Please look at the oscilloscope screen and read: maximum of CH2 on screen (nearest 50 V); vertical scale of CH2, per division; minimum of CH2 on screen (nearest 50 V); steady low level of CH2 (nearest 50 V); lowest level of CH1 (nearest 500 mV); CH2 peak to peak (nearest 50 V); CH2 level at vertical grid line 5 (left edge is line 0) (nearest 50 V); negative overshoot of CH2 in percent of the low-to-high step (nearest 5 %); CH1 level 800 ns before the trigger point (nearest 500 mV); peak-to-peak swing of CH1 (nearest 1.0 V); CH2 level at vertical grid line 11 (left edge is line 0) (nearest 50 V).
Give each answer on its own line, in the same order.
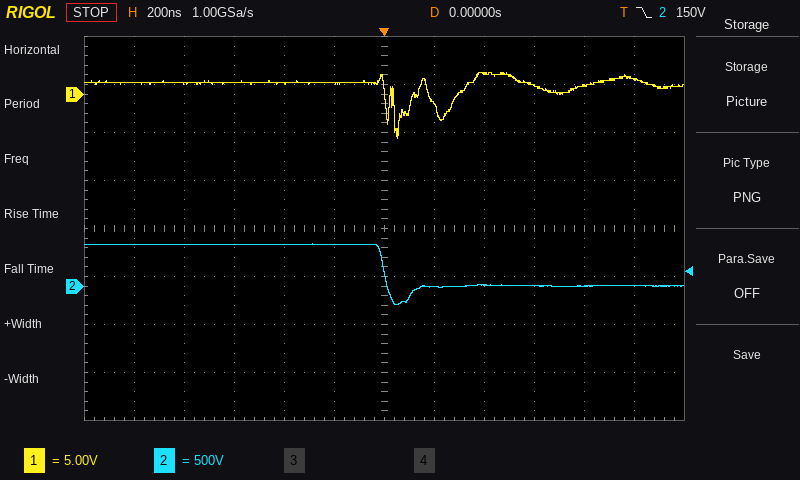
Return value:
450 V
500 V
-200 V
0 V
-4.5 V
650 V
450 V
45 %
1.0 V
7.0 V
0 V
